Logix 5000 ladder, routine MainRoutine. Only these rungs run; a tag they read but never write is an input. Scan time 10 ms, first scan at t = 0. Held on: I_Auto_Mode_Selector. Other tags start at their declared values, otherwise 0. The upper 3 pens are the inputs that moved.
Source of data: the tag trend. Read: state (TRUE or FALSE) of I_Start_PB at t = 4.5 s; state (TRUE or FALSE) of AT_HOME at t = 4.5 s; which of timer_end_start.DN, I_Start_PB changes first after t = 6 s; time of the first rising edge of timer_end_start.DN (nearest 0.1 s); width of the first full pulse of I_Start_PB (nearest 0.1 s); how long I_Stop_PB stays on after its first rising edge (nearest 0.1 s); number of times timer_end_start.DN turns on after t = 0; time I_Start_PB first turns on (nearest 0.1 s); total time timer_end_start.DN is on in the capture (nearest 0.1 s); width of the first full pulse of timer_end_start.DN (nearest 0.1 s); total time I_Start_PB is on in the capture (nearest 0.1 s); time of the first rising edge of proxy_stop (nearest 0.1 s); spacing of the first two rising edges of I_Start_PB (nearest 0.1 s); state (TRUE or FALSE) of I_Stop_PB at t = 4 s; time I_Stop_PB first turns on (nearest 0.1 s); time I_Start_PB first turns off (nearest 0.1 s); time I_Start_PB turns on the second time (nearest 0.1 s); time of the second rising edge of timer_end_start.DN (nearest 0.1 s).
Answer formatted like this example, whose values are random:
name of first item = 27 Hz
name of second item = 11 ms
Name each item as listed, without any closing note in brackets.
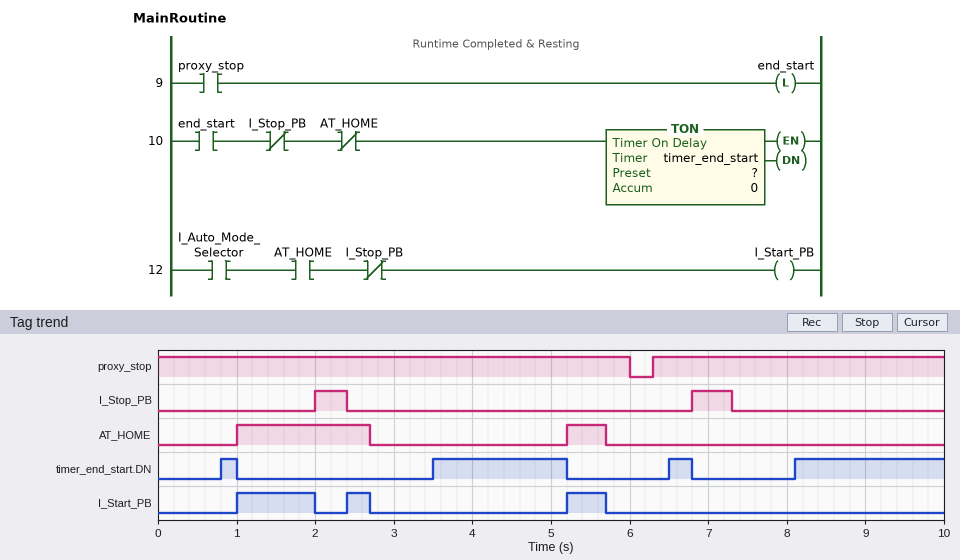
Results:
state (TRUE or FALSE) of I_Start_PB at t = 4.5 s = FALSE
state (TRUE or FALSE) of AT_HOME at t = 4.5 s = FALSE
which of timer_end_start.DN, I_Start_PB changes first after t = 6 s = timer_end_start.DN
time of the first rising edge of timer_end_start.DN = 0.8 s
width of the first full pulse of I_Start_PB = 1.0 s
how long I_Stop_PB stays on after its first rising edge = 0.4 s
number of times timer_end_start.DN turns on after t = 0 = 4
time I_Start_PB first turns on = 1.0 s
total time timer_end_start.DN is on in the capture = 4.1 s
width of the first full pulse of timer_end_start.DN = 0.2 s
total time I_Start_PB is on in the capture = 1.8 s
time of the first rising edge of proxy_stop = 6.3 s
spacing of the first two rising edges of I_Start_PB = 1.4 s
state (TRUE or FALSE) of I_Stop_PB at t = 4 s = FALSE
time I_Stop_PB first turns on = 2.0 s
time I_Start_PB first turns off = 2.0 s
time I_Start_PB turns on the second time = 2.4 s
time of the second rising edge of timer_end_start.DN = 3.5 s
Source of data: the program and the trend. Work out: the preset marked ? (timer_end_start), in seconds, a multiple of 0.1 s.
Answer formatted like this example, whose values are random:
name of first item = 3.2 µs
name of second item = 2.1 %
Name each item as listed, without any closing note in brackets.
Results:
the preset marked ? (timer_end_start), in seconds, a multiple of 0.1 s = 0.8 s
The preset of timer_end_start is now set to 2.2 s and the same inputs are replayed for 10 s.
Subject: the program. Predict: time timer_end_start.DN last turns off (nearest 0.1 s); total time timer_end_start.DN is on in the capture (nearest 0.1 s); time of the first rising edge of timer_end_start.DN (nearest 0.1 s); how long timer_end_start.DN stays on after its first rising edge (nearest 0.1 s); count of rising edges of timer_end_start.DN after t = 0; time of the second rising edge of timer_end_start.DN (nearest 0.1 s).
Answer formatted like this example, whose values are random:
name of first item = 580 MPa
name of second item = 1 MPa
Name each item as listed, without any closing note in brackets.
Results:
time timer_end_start.DN last turns off = 5.2 s
total time timer_end_start.DN is on in the capture = 0.8 s
time of the first rising edge of timer_end_start.DN = 4.9 s
how long timer_end_start.DN stays on after its first rising edge = 0.3 s
count of rising edges of timer_end_start.DN after t = 0 = 2
time of the second rising edge of timer_end_start.DN = 9.5 s
